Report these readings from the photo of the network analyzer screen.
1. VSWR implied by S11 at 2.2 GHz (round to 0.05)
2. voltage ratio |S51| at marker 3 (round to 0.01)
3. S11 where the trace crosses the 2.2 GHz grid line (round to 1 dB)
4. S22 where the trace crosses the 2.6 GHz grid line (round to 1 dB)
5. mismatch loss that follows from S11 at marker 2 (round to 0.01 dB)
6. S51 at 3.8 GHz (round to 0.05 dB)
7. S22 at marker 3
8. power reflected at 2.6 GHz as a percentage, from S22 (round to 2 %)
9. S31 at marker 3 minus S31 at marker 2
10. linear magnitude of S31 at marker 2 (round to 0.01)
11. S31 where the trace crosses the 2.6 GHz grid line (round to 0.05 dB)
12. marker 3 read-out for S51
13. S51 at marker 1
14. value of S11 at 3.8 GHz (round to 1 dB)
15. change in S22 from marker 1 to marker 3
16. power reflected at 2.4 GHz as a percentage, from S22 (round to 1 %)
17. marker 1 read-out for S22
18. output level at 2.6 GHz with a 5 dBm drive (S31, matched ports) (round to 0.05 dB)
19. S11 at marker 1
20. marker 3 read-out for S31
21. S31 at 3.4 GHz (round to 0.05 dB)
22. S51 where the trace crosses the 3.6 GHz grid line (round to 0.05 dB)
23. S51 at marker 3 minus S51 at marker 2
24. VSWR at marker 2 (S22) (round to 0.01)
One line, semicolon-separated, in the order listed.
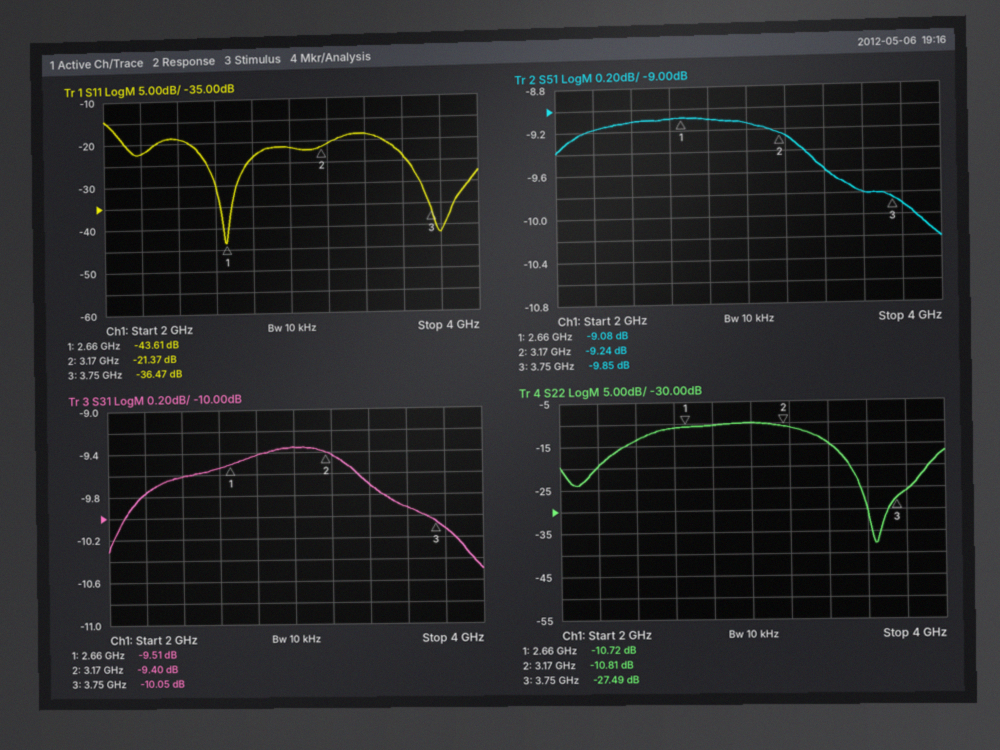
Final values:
1.15; 0.32; -22 dB; -11 dB; 0.03 dB; -9.90 dB; -27.49 dB; 8 %; -0.65 dB; 0.34; -9.55 dB; -9.85 dB; -9.08 dB; -42 dB; -16.77 dB; 4 %; -10.72 dB; -4.55 dBm; -43.61 dB; -10.05 dB; -9.70 dB; -9.80 dB; -0.61 dB; 1.81
